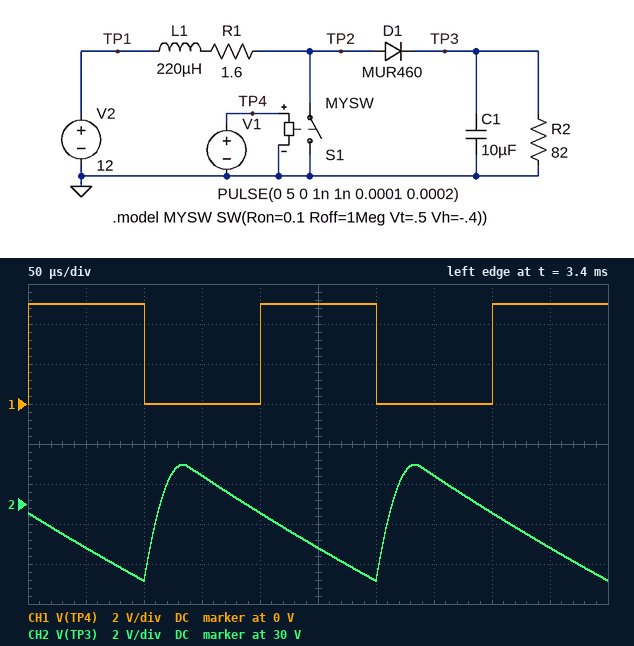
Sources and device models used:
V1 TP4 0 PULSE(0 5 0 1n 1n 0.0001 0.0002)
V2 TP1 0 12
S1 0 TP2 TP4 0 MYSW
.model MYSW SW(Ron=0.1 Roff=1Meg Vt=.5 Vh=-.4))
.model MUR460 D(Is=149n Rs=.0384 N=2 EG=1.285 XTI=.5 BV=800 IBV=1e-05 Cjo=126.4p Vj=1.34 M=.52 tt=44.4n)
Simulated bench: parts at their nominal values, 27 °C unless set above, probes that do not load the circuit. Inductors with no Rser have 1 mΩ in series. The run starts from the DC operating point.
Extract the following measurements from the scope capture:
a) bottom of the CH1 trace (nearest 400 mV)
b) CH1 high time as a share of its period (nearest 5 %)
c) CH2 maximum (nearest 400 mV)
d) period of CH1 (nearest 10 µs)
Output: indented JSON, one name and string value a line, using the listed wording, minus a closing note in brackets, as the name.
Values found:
{
  "bottom of the CH1 trace": "0 V",
  "CH1 high time as a share of its period": "50 %",
  "CH2 maximum": "32.0 V",
  "period of CH1": "200 µs"
}
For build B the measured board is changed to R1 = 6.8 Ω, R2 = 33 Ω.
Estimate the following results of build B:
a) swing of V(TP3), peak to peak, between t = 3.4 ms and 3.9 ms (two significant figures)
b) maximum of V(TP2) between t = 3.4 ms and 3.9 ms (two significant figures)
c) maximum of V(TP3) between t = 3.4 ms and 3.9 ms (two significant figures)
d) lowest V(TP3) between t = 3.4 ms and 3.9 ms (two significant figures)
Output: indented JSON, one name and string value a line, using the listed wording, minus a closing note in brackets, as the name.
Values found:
{
  "swing of V(TP3), peak to peak, between t = 3.4 ms and 3.9 ms": "3.3 V",
  "maximum of V(TP2) between t = 3.4 ms and 3.9 ms": "12 V",
  "maximum of V(TP3) between t = 3.4 ms and 3.9 ms": "11 V",
  "lowest V(TP3) between t = 3.4 ms and 3.9 ms": "7.9 V"
}
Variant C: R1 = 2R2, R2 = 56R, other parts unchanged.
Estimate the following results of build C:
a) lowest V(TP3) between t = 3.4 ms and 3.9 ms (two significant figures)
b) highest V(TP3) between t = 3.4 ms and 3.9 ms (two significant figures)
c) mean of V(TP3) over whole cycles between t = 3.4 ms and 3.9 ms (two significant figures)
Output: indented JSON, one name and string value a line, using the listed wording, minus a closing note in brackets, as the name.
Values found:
{
  "lowest V(TP3) between t = 3.4 ms and 3.9 ms": "19 V",
  "highest V(TP3) between t = 3.4 ms and 3.9 ms": "25 V",
  "mean of V(TP3) over whole cycles between t = 3.4 ms and 3.9 ms": "22 V"
}
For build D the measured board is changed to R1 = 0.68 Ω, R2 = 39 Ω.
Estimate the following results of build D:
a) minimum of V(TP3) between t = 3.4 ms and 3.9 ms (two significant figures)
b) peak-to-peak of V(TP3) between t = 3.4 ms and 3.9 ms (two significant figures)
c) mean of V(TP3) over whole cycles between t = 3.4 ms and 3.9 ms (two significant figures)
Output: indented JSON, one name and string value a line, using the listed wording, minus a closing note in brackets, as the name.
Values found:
{
  "minimum of V(TP3) between t = 3.4 ms and 3.9 ms": "21 V",
  "peak-to-peak of V(TP3) between t = 3.4 ms and 3.9 ms": "9.7 V",
  "mean of V(TP3) over whole cycles between t = 3.4 ms and 3.9 ms": "26 V"
}
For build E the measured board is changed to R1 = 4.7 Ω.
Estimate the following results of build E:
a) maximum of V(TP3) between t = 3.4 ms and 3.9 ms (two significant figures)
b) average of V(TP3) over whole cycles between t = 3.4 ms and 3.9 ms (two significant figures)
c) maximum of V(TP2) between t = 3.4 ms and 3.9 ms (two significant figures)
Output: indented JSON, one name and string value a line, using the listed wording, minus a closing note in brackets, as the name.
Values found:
{
  "maximum of V(TP3) between t = 3.4 ms and 3.9 ms": "19 V",
  "average of V(TP3) over whole cycles between t = 3.4 ms and 3.9 ms": "17 V",
  "maximum of V(TP2) between t = 3.4 ms and 3.9 ms": "20 V"
}
